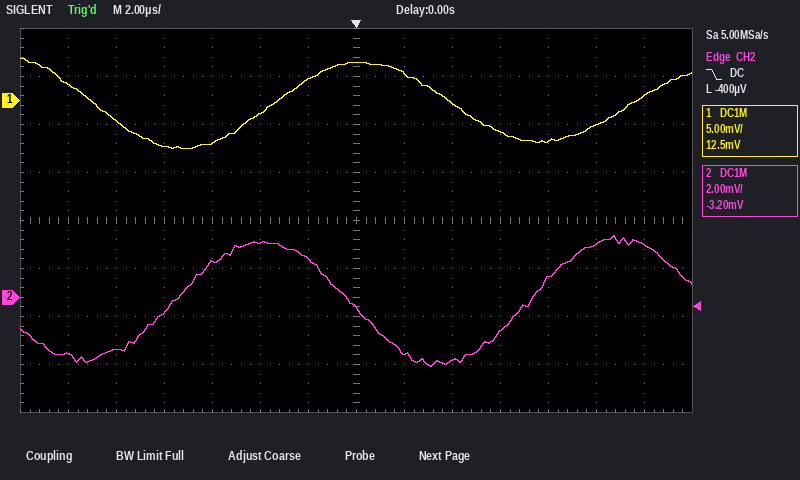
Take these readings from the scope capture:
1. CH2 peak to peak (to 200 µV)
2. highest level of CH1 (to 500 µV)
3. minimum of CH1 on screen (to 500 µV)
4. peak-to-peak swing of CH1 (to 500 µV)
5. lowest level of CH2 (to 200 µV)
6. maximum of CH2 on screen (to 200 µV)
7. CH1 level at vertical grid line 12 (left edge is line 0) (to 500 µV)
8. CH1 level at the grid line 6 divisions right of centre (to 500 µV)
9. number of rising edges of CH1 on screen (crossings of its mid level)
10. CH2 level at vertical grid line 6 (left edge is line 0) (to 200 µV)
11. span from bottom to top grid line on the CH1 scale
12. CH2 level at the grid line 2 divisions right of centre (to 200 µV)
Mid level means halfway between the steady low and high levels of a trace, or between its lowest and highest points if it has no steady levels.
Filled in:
5.4 mV
4.5 mV
-5.0 mV
9.5 mV
-2.8 mV
2.6 mV
-2.5 mV
500 µV
2
1.6 mV
40 mV
-2.6 mV
